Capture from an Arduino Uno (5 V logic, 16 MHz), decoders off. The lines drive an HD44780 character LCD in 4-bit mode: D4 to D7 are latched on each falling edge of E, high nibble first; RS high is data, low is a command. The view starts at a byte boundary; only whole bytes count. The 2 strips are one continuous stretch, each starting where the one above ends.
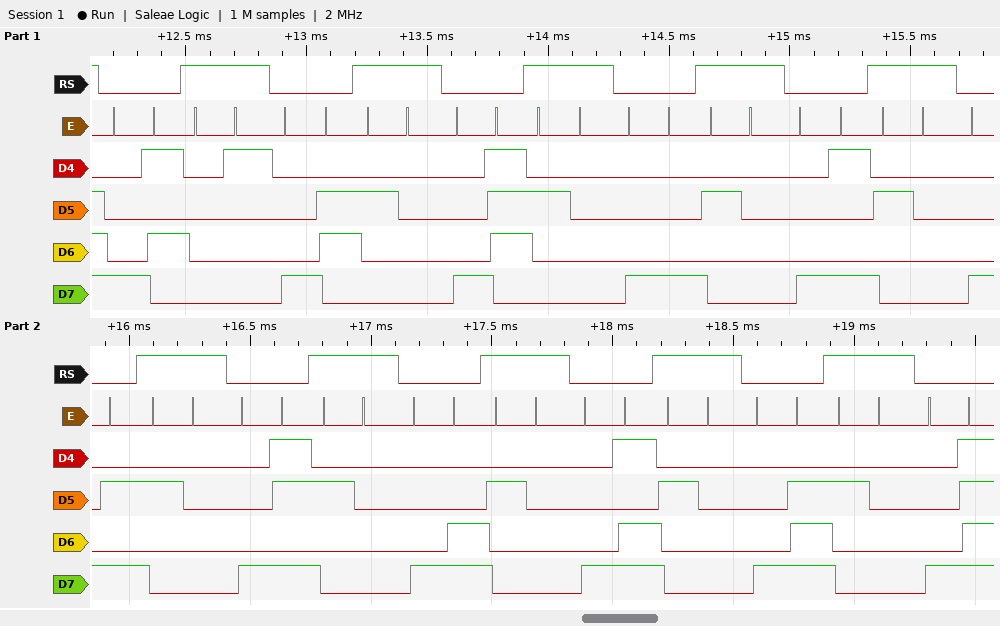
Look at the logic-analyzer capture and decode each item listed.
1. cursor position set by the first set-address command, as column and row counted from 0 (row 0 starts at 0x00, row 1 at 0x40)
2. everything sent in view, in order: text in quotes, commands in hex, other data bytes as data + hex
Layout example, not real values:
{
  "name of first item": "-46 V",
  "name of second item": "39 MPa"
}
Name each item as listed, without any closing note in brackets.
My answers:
{
  "cursor position set by the first set-address command, as column and row counted from 0": "column 5, row 0",
  "everything sent in view, in order: text in quotes, commands in hex, other data bytes as data + hex": "0x85 data 01 0x86 \" \" 0x87 \" \" 0x88 \" \" 0x89 \" \" 0x8A \" \" 0x8B \" \" 0x8C \" \" 0x8D \" \" 0x8E \" \" 0x8F"
}
